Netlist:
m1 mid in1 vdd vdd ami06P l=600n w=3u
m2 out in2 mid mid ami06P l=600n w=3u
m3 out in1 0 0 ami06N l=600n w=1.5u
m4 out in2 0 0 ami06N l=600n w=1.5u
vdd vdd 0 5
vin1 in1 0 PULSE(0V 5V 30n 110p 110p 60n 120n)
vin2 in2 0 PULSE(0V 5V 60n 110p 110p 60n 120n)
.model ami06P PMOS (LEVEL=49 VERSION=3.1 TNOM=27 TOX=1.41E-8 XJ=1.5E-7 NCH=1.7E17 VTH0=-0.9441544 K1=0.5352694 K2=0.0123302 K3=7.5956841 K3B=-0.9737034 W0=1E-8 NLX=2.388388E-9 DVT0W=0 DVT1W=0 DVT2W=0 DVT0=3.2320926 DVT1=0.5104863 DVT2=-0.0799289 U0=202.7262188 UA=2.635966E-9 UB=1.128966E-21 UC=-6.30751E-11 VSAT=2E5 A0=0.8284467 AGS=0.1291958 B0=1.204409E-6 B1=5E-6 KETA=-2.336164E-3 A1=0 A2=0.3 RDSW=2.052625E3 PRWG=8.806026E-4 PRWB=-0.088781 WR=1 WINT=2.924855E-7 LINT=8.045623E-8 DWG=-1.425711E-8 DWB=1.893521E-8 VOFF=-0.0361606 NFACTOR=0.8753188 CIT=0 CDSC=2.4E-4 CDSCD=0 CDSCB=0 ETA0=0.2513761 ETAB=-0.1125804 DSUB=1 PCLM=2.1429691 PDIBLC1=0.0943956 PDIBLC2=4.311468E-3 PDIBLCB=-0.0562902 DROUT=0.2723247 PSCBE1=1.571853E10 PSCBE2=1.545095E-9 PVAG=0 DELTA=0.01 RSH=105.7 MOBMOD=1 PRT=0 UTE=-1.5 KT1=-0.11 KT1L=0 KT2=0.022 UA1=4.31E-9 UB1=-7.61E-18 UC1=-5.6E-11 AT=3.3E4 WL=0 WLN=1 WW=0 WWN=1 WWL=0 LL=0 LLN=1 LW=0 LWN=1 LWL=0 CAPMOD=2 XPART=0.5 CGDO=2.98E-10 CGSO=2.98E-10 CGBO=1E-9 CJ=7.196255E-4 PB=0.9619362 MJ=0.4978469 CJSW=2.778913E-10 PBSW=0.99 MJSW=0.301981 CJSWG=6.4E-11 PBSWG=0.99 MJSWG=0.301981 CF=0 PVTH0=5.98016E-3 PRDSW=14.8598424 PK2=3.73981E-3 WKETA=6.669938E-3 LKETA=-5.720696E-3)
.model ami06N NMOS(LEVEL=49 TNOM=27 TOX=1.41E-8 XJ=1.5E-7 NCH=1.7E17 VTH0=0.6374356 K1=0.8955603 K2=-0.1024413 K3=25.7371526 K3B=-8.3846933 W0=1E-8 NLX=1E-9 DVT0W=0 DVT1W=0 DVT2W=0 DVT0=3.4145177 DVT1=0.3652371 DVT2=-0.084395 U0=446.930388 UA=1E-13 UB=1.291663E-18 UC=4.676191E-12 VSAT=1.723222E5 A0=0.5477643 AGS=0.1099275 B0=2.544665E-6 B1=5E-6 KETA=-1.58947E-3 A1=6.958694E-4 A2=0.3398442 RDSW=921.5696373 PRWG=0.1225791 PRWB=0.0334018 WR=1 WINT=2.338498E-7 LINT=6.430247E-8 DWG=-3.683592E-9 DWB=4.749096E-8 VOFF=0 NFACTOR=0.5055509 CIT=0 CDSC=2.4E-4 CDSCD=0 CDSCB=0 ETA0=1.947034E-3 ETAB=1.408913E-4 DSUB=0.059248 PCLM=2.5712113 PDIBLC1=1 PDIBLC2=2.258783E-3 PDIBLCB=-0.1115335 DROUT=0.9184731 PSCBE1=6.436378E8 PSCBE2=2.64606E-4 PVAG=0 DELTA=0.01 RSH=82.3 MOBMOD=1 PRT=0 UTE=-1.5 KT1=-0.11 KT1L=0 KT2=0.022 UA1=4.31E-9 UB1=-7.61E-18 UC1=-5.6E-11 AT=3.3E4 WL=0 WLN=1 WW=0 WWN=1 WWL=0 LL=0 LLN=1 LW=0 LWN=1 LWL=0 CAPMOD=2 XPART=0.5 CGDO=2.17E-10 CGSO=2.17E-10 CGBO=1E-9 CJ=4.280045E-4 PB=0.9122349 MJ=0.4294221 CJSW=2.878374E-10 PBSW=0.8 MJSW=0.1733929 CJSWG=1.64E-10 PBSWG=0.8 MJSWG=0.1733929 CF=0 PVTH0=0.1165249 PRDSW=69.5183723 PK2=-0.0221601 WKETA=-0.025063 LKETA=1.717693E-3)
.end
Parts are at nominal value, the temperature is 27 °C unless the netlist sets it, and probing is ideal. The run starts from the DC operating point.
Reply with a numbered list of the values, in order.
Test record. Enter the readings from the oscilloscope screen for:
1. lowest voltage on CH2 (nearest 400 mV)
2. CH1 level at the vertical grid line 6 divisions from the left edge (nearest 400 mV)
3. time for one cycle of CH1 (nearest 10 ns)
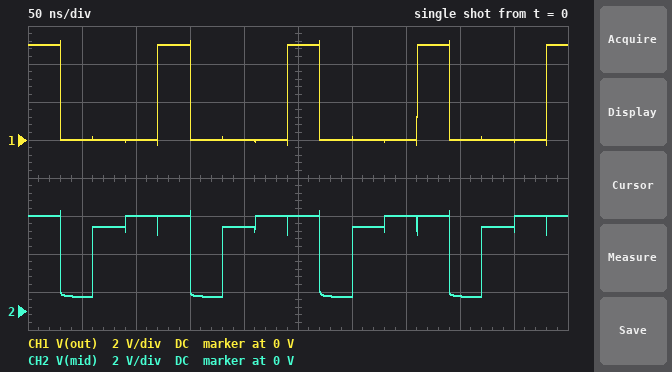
1. 800 mV
2. 0 V
3. 120 ns
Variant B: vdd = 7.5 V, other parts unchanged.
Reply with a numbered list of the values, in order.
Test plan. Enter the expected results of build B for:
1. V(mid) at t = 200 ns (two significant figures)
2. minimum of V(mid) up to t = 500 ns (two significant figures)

1. 6.8 V
2. 2.7 V
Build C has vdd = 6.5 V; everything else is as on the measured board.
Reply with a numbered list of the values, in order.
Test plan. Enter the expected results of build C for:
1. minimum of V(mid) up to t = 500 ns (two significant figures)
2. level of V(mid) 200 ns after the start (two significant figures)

1. 1.7 V
2. 6.2 V
